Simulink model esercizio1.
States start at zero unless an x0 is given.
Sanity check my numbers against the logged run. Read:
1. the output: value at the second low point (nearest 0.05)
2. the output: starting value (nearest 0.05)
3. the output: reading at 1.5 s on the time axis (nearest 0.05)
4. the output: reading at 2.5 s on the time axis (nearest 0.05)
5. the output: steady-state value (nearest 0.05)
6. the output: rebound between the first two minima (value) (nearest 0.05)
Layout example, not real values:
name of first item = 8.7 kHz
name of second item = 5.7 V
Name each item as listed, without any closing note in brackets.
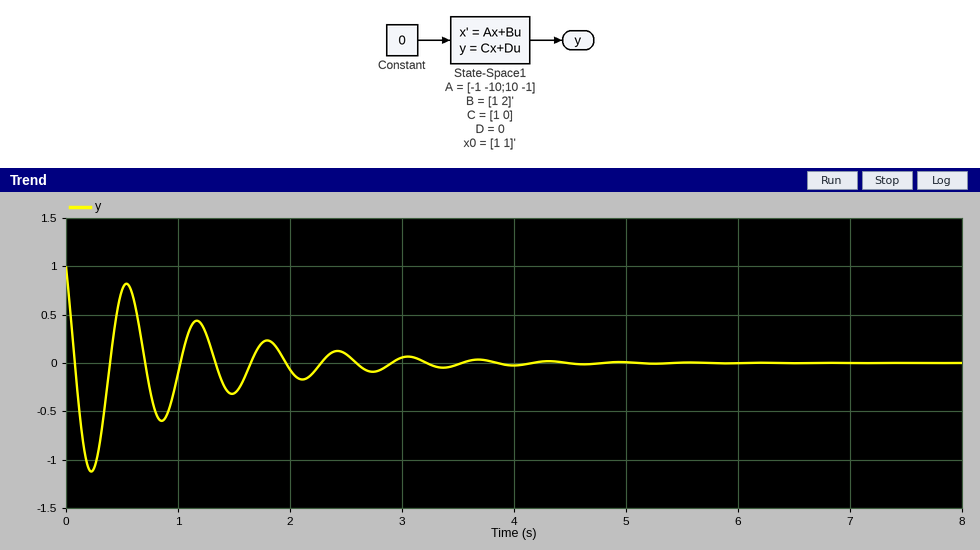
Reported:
the output: value at the second low point = -0.60
the output: starting value = 1.00
the output: reading at 1.5 s on the time axis = -0.30
the output: reading at 2.5 s on the time axis = 0.10
the output: steady-state value = 0.00
the output: rebound between the first two minima (value) = 0.80
